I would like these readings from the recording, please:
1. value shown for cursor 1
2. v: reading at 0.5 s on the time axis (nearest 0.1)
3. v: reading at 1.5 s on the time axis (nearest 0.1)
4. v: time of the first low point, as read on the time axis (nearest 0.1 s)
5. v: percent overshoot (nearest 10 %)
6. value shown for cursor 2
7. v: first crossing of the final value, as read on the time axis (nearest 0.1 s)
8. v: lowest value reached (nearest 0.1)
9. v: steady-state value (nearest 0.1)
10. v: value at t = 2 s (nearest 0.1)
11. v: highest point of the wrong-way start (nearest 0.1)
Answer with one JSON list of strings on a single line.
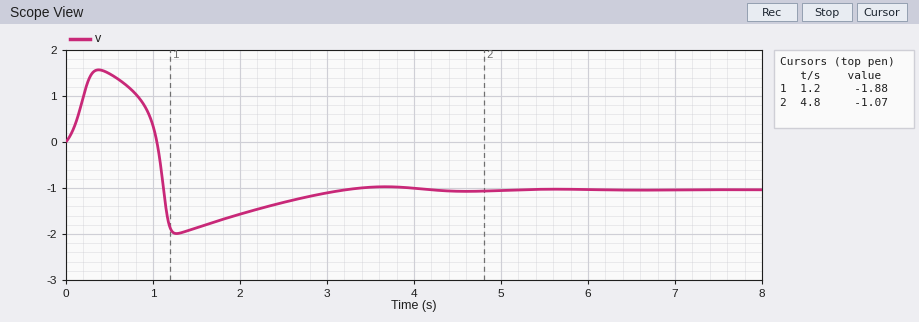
["-1.88", "1.5", "-1.9", "1.3 s", "90 %", "-1.07", "1.1 s", "-2.0", "-1.0", "-1.6", "1.6"]
